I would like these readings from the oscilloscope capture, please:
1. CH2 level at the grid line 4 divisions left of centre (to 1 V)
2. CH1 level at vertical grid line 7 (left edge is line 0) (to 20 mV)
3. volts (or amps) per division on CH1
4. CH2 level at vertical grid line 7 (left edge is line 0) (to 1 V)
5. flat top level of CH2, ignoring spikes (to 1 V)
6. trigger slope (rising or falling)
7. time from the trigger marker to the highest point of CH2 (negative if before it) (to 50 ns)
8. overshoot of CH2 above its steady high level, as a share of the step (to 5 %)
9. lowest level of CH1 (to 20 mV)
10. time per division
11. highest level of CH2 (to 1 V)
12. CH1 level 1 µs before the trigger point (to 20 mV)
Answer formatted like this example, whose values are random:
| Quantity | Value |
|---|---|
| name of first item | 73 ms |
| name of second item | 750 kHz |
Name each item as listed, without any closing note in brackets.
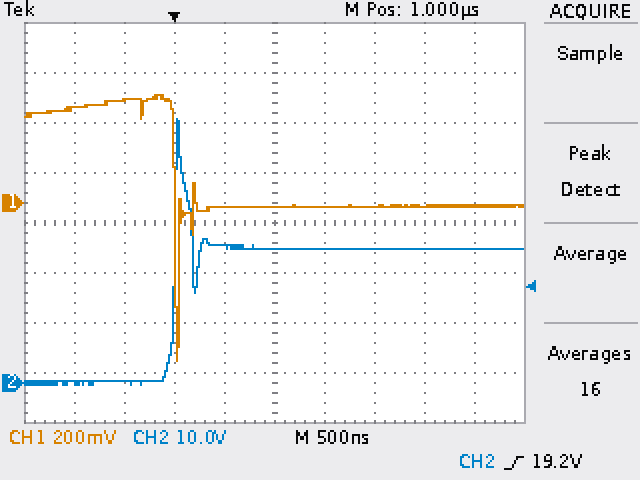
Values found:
| Quantity | Value |
|---|---|
| CH2 level at the grid line 4 divisions left of centre | 0 V |
| CH1 level at vertical grid line 7 (left edge is line 0) | -20 mV |
| volts (or amps) per division on CH1 | 200 mV |
| CH2 level at vertical grid line 7 (left edge is line 0) | 27 V |
| flat top level of CH2, ignoring spikes | 27 V |
| trigger slope | rising |
| time from the trigger marker to the highest point of CH2 (negative if before it) | +50 ns |
| overshoot of CH2 above its steady high level, as a share of the step | 100 % |
| lowest level of CH1 | -640 mV |
| time per division | 500 ns |
| highest level of CH2 | 53 V |
| CH1 level 1 µs before the trigger point | 380 mV |
